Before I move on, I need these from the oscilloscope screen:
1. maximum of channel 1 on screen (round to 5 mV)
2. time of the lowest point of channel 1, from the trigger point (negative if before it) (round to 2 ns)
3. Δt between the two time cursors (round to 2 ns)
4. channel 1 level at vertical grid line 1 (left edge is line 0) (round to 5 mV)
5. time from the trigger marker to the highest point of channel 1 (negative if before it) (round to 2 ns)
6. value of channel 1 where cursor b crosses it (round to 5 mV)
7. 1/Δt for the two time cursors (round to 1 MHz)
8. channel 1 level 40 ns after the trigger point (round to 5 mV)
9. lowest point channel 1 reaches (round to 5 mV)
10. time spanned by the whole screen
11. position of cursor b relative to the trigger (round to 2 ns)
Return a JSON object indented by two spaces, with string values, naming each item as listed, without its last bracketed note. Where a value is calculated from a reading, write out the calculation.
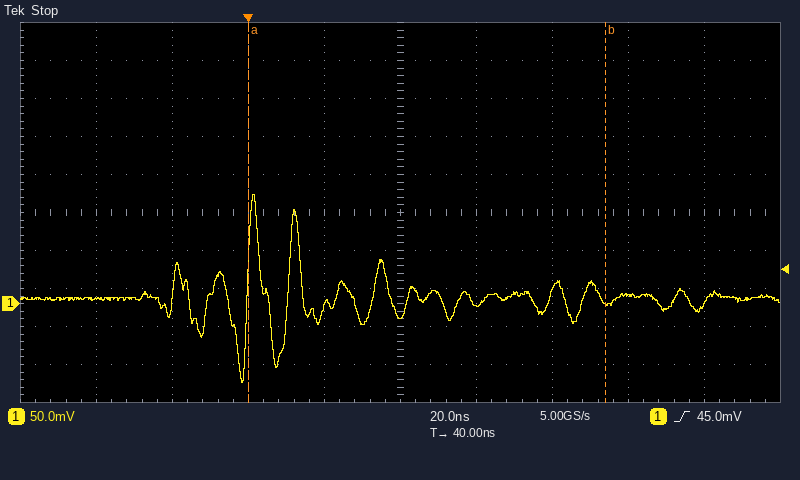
{
  "maximum of channel 1 on screen": "145 mV",
  "time of the lowest point of channel 1, from the trigger point (negative if before it)": "-2 ns",
  "Δt between the two time cursors": "94 ns",
  "channel 1 level at vertical grid line 1 (left edge is line 0)": "5 mV",
  "time from the trigger marker to the highest point of channel 1 (negative if before it)": "+2 ns",
  "value of channel 1 where cursor b crosses it": "0 mV",
  "1/Δt for the two time cursors": "1 / 94 ns ≈ 11 MHz",
  "channel 1 level 40 ns after the trigger point": "-15 mV",
  "lowest point channel 1 reaches": "-105 mV",
  "time spanned by the whole screen": "200 ns",
  "position of cursor b relative to the trigger": "+94 ns"
}
